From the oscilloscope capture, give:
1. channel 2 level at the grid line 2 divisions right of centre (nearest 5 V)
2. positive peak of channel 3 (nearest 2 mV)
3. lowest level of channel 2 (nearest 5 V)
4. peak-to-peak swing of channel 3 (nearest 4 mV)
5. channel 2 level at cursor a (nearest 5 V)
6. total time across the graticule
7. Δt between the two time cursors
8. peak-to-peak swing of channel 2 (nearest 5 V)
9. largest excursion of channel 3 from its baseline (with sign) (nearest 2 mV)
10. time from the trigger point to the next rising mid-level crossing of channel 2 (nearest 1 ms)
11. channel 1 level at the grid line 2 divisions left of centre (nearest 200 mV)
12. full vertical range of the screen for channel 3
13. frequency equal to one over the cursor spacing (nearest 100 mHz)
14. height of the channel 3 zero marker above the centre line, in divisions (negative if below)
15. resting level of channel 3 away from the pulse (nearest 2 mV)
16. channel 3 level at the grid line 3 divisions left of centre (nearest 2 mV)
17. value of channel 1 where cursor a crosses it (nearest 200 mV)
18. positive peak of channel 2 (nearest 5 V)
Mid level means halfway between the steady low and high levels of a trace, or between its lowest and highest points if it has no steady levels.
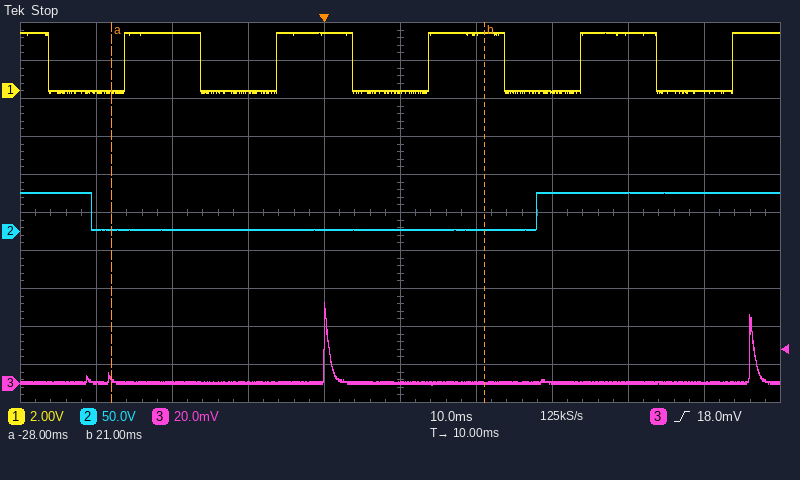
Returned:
50 V
42 mV
0 V
44 mV
0 V
100 ms
49 ms
50 V
+42 mV
28 ms
0.0 V
200 mV
20.4 Hz
-4.5 div
0 mV
0 mV
0.0 V
50 V
